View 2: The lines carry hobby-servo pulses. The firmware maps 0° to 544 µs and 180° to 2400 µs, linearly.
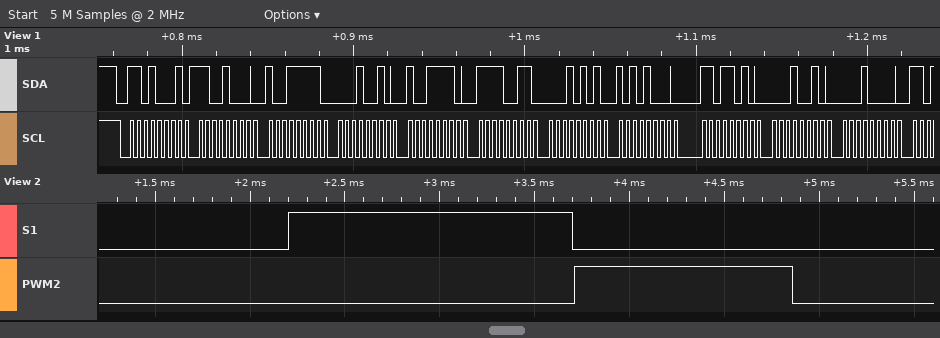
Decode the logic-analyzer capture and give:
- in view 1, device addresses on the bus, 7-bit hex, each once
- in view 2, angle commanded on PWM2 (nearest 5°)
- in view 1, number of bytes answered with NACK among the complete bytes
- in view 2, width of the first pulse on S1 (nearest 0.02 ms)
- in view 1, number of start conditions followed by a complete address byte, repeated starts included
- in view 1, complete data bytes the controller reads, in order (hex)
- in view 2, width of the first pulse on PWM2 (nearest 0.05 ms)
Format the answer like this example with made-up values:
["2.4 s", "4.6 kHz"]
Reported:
["0x68", "60°", "0", "1.50 ms", "1", "C8 9F 12 9E F3 15 A8 DA 12 10", "1.15 ms"]
